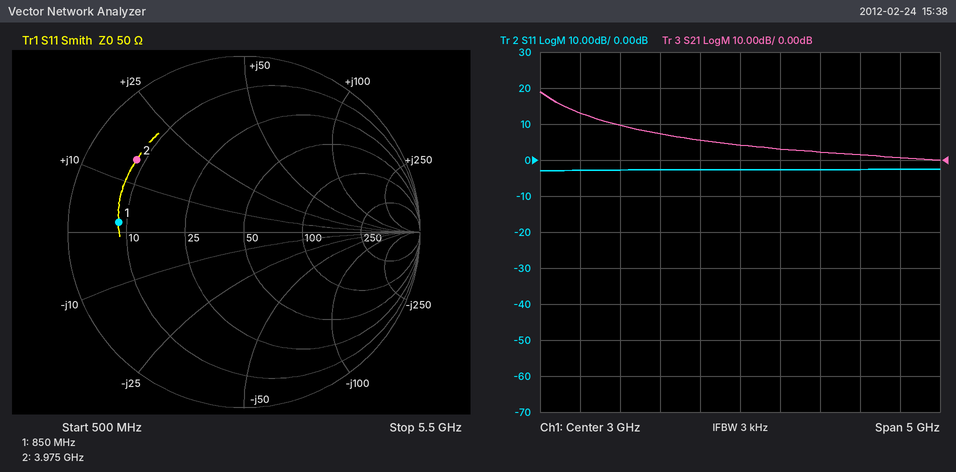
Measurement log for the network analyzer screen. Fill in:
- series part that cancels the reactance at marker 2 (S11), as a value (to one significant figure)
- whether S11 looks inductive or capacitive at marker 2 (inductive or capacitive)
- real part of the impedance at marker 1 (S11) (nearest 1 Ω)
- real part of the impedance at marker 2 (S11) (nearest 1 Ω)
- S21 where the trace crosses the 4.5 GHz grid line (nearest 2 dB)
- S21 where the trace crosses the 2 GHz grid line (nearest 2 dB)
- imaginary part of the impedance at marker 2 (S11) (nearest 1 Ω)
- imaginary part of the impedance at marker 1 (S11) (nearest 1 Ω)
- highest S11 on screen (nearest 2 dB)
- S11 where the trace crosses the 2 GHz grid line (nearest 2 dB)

3 pF
inductive
8 Ω
8 Ω
2 dB
8 dB
+15 Ω
+2 Ω
-2 dB
-2 dB
